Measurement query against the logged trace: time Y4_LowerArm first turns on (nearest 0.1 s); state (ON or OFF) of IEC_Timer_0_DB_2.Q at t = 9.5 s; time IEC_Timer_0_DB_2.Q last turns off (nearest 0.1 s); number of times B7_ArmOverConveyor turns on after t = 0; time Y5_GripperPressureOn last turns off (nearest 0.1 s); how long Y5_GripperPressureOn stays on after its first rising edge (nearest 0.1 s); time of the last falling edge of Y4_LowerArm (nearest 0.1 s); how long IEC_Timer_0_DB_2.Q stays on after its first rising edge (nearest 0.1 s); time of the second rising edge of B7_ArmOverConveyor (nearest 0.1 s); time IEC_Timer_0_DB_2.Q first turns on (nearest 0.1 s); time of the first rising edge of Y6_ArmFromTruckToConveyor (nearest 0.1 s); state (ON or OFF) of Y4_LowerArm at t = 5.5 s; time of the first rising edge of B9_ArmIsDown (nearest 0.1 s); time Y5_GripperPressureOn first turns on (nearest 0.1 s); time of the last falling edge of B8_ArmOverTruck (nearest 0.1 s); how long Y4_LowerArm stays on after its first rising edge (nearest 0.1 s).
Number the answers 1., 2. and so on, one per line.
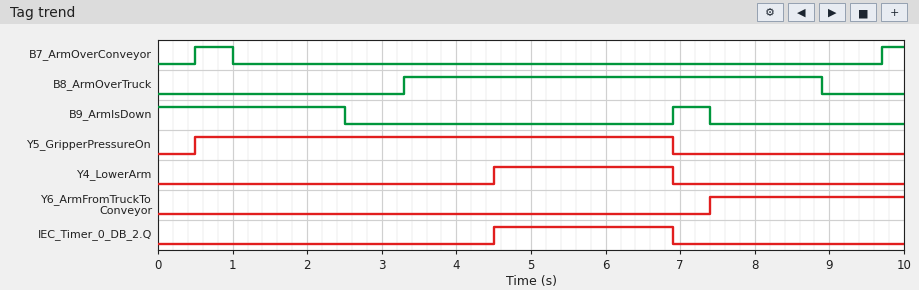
1. 4.5 s
2. OFF
3. 6.9 s
4. 2
5. 6.9 s
6. 6.4 s
7. 6.9 s
8. 2.4 s
9. 9.7 s
10. 4.5 s
11. 7.4 s
12. ON
13. 6.9 s
14. 0.5 s
15. 8.9 s
16. 2.4 s
